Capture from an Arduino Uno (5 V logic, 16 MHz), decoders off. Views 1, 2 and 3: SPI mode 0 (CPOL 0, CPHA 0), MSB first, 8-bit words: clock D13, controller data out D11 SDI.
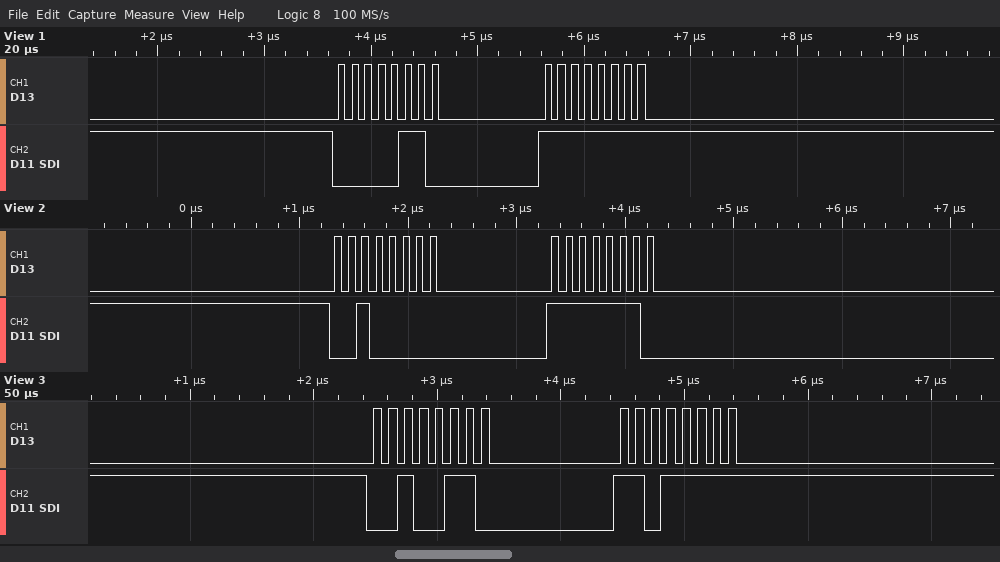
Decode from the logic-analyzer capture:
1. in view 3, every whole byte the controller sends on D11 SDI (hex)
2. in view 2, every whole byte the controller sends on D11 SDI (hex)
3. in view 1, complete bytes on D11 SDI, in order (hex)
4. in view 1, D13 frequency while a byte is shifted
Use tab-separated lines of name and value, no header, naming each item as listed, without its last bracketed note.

in view 3, every whole byte the controller sends on D11 SDI	26 DF
in view 2, every whole byte the controller sends on D11 SDI	20 FE
in view 1, complete bytes on D11 SDI, in order	06 FF
in view 1, D13 frequency while a byte is shifted	8 MHz
